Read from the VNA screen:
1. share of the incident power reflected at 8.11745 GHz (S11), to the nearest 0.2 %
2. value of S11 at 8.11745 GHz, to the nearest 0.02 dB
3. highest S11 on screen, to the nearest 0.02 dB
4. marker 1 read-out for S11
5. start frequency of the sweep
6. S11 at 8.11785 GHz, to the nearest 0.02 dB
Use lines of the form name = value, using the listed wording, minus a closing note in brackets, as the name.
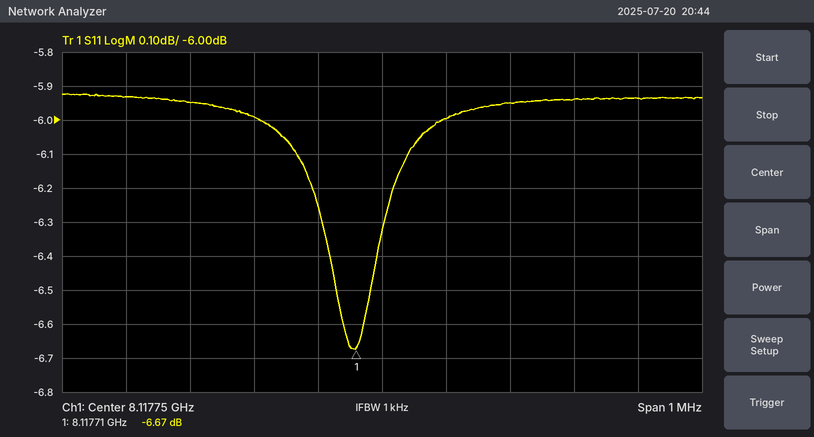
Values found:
share of the incident power reflected at 8.11745 GHz (S11), to the nearest 0.2 % = 25.4 %
value of S11 at 8.11745 GHz, to the nearest 0.02 dB = -5.94 dB
highest S11 on screen, to the nearest 0.02 dB = -5.92 dB
marker 1 read-out for S11 = -6.67 dB
start frequency of the sweep = 8.11725 GHz
S11 at 8.11785 GHz, to the nearest 0.02 dB = -6.00 dB
